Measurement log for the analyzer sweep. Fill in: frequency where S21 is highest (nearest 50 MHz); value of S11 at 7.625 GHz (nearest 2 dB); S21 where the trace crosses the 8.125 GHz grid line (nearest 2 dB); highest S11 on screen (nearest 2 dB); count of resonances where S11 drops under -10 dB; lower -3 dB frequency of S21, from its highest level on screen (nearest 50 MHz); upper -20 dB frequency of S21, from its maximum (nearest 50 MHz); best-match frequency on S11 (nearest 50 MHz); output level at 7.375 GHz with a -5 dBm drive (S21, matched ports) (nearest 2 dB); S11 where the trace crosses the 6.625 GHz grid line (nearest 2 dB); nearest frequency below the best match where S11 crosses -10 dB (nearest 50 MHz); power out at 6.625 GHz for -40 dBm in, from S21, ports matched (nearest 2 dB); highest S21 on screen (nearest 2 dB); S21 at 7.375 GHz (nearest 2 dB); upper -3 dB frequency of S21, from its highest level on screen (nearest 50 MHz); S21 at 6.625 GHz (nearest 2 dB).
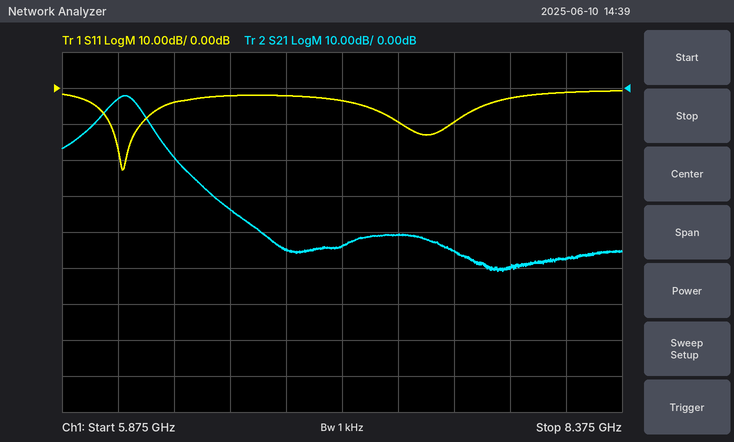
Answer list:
6.15 GHz
-10 dB
-48 dB
0 dB
2
6.10 GHz
6.40 GHz
6.15 GHz
-46 dBm
-2 dB
6.10 GHz
-74 dBm
-2 dB
-40 dB
6.20 GHz
-34 dB
